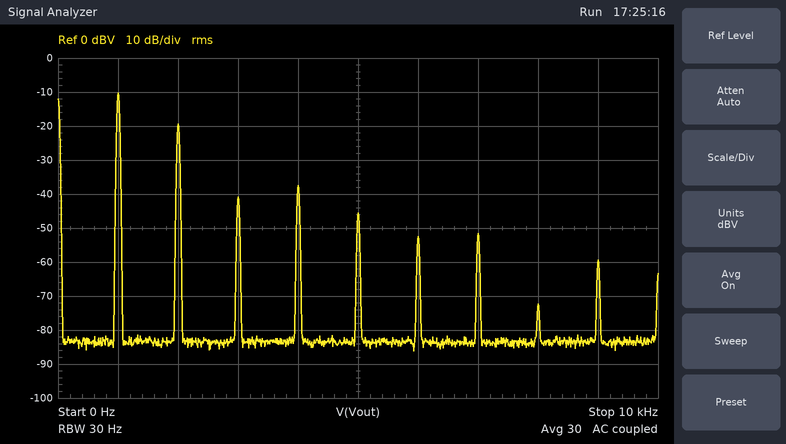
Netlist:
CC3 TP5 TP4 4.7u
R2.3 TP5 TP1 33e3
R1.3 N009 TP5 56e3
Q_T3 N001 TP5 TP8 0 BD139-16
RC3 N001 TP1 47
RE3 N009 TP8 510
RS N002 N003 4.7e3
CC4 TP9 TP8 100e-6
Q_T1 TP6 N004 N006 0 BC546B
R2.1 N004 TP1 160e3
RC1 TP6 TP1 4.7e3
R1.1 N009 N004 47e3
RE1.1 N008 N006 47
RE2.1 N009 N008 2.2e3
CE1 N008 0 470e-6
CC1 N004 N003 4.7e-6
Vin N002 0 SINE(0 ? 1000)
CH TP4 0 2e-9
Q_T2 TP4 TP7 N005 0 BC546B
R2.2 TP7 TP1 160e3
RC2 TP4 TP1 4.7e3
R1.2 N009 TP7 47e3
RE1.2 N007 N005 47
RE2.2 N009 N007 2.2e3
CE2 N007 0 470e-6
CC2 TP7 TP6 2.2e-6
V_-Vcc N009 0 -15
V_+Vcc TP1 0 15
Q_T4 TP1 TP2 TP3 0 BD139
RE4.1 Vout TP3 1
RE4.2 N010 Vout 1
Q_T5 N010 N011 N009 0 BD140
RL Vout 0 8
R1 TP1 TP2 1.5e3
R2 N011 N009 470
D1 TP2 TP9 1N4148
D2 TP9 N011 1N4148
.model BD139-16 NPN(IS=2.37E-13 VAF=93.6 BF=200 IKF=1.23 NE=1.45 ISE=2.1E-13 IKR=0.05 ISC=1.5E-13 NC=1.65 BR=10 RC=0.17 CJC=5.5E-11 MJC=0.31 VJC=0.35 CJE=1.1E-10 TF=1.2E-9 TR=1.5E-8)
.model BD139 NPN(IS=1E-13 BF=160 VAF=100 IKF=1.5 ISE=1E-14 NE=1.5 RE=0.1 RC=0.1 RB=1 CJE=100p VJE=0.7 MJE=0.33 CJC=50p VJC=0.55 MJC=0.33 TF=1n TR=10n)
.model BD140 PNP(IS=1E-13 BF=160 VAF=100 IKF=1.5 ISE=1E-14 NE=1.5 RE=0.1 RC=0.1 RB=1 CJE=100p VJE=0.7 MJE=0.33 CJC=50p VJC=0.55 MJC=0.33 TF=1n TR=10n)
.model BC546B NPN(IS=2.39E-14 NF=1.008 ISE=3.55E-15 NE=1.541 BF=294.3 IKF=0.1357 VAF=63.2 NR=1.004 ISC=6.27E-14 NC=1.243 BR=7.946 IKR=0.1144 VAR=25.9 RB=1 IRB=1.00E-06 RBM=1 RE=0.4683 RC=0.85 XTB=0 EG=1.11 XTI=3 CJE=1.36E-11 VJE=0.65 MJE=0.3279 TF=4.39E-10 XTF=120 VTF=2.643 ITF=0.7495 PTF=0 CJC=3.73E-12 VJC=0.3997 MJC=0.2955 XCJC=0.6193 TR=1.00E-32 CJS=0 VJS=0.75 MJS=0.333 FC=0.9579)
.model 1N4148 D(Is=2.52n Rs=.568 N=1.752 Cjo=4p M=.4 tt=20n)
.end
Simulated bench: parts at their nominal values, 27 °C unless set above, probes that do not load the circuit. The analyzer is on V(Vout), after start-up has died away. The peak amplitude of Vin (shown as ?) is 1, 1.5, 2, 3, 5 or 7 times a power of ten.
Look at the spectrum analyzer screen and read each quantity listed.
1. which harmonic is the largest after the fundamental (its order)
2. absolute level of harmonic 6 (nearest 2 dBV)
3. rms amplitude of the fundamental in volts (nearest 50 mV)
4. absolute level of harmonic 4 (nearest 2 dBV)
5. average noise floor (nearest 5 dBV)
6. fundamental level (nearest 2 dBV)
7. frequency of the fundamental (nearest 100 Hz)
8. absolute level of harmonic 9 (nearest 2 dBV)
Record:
2
-52 dBV
300 mV
-38 dBV
-85 dBV
-10 dBV
1.0 kHz
-60 dBV
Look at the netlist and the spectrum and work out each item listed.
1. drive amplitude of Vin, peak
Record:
500 µV
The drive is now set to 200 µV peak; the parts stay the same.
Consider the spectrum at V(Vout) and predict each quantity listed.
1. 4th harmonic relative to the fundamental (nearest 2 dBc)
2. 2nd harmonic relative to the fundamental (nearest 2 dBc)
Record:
-58 dBc
-20 dBc
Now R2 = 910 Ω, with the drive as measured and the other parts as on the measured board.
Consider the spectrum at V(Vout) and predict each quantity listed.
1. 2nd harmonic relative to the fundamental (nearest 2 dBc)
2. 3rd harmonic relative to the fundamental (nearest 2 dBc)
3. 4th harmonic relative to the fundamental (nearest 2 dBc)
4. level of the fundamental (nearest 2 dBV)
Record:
-16 dBc
-24 dBc
-36 dBc
-6 dBV
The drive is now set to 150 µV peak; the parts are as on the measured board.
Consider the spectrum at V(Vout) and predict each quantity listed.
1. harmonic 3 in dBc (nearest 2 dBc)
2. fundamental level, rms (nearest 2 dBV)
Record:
-40 dBc
-18 dBV
